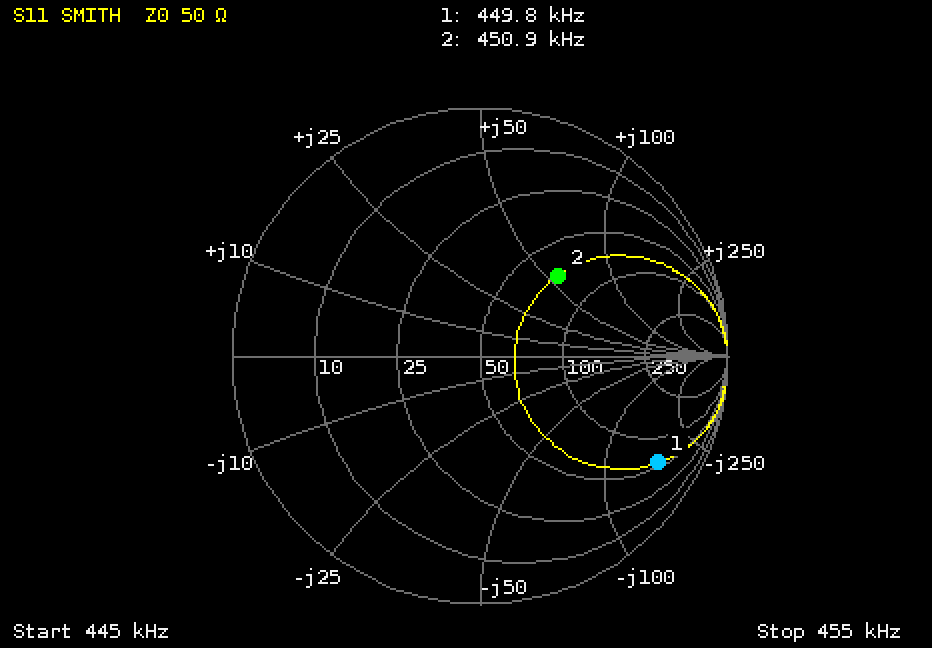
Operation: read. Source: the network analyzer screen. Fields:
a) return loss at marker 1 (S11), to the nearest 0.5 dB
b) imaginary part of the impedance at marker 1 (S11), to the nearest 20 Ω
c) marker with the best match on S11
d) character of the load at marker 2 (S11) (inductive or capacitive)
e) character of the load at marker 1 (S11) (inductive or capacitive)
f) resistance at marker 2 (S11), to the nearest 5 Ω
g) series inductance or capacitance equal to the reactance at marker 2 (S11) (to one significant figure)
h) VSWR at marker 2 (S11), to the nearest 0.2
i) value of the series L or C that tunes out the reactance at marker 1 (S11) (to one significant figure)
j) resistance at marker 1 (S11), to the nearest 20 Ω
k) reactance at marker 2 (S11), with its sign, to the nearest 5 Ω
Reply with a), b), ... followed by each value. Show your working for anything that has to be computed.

a) 1.5 dB
b) -160 Ω
c) marker 2
d) inductive
e) capacitive
f) 70 Ω
g) L = 55 Ω/(2π × 450.9 kHz) ≈ 19.4 µH, so 20 µH to one significant figure
h) 2.6
i) L = 160 Ω/(2π × 449.8 kHz) ≈ 56.6 µH, so 60 µH to one significant figure
j) 60 Ω
k) +55 Ω
